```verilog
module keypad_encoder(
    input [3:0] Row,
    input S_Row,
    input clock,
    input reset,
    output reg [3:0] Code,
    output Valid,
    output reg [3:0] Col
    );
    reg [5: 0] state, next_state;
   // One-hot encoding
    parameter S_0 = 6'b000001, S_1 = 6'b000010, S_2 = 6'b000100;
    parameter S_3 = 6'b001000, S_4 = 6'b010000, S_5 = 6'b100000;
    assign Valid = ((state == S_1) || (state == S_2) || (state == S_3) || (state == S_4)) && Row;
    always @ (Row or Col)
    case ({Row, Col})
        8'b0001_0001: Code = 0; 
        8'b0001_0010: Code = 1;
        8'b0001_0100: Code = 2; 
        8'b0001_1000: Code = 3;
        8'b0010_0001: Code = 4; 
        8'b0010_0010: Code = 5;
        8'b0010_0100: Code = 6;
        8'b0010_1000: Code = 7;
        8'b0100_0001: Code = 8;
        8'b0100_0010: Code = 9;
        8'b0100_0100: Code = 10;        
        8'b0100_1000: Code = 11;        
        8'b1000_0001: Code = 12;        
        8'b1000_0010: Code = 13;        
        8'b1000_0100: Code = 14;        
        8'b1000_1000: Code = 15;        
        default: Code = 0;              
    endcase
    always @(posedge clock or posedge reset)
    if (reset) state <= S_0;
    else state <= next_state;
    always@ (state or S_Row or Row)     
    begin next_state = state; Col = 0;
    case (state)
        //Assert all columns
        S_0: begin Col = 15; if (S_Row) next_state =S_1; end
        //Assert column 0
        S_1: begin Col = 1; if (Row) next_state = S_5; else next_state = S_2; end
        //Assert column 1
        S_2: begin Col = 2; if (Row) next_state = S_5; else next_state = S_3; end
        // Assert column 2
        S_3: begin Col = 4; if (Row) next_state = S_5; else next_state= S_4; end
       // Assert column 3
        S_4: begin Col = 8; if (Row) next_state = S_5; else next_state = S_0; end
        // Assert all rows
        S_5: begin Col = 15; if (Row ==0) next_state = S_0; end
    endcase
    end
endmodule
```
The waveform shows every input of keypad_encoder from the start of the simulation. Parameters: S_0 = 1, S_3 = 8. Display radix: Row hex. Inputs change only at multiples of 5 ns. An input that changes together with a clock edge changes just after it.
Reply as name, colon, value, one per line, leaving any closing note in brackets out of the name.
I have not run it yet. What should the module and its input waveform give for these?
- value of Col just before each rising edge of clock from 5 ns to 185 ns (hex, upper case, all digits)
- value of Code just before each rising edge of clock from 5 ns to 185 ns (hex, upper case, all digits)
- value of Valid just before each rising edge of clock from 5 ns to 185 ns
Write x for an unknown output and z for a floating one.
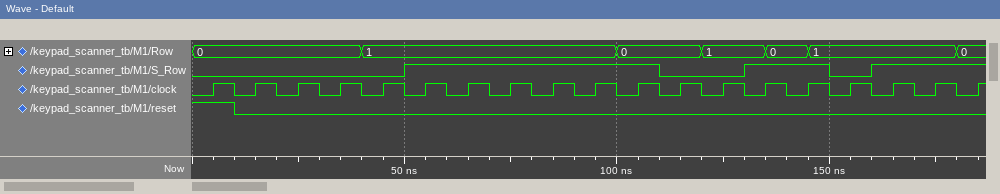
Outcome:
value of Col just before each rising edge of clock from 5 ns to 185 ns: F, F, F, F, F, F, 1, F, F, F, F, F, F, F, 1, 2, F, F, F
value of Code just before each rising edge of clock from 5 ns to 185 ns: 0, 0, 0, 0, 0, 0, 0, 0, 0, 0, 0, 0, 0, 0, 0, 1, 0, 0, 0
value of Valid just before each rising edge of clock from 5 ns to 185 ns: 0 0 0 0 0 0 1 0 0 0 0 0 0 0 0 1 0 0 0
